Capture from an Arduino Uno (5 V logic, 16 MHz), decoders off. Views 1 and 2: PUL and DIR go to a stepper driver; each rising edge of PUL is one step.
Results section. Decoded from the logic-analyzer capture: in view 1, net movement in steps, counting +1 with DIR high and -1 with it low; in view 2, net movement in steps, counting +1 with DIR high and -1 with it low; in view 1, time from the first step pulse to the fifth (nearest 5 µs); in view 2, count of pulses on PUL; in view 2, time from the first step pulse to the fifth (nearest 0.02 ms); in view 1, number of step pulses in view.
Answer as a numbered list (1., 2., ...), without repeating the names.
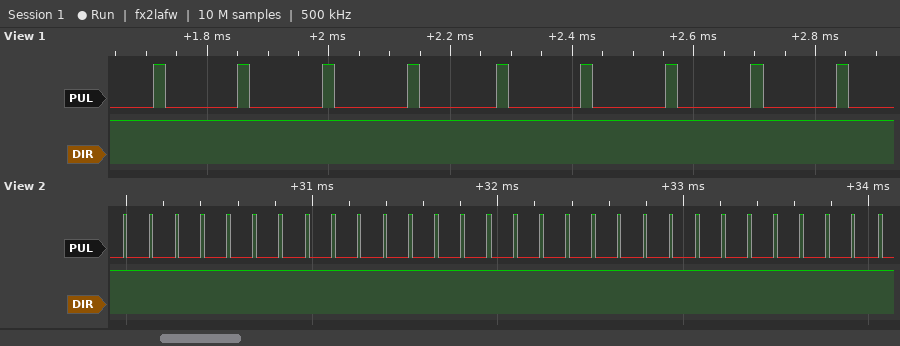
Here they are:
1. +9
2. +30
3. 565 µs
4. 30
5. 0.56 ms
6. 9
